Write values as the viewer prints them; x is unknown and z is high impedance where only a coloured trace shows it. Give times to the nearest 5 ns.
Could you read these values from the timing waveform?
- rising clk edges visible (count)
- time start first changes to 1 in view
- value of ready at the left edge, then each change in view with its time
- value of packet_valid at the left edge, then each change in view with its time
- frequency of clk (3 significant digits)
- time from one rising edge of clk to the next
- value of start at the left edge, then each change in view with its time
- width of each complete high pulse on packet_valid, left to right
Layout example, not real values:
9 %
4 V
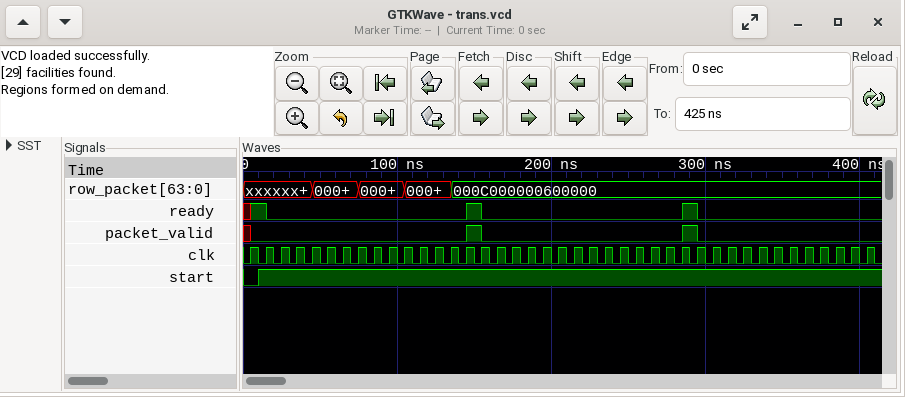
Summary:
41
10 ns
x, 1 at 5 ns, 0 at 15 ns, 1 at 145 ns, 0 at 155 ns, 1 at 285 ns, 0 at 295 ns
x, 0 at 5 ns, 1 at 145 ns, 0 at 155 ns, 1 at 285 ns, 0 at 295 ns
100 MHz
10 ns
0, 1 at 10 ns
10 ns, 10 ns
